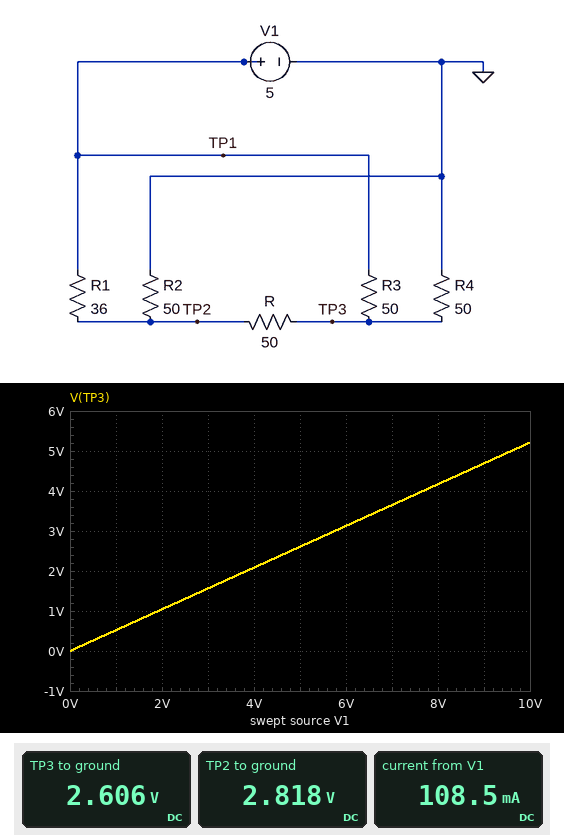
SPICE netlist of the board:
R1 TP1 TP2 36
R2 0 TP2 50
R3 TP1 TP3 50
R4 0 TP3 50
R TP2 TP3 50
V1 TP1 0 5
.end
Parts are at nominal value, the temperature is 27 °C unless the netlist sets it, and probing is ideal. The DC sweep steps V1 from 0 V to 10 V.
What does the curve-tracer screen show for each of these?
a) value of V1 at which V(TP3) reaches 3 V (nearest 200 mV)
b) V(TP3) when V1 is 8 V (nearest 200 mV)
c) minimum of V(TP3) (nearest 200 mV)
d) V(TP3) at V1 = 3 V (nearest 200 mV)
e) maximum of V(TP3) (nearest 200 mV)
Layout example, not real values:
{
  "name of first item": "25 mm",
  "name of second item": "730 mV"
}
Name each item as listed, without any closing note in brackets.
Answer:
{
  "value of V1 at which V(TP3) reaches 3 V": "5.8 V",
  "V(TP3) when V1 is 8 V": "4.2 V",
  "minimum of V(TP3)": "0 V",
  "V(TP3) at V1 = 3 V": "1.6 V",
  "maximum of V(TP3)": "5.2 V"
}
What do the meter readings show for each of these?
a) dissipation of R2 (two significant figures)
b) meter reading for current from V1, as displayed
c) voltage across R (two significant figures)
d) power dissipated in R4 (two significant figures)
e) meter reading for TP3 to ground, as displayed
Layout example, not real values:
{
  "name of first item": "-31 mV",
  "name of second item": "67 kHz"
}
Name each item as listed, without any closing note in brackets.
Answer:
{
  "dissipation of R2": "160 mW",
  "meter reading for current from V1, as displayed": "108.5 mA",
  "voltage across R": "210 mV",
  "power dissipated in R4": "140 mW",
  "meter reading for TP3 to ground, as displayed": "2.606 V"
}
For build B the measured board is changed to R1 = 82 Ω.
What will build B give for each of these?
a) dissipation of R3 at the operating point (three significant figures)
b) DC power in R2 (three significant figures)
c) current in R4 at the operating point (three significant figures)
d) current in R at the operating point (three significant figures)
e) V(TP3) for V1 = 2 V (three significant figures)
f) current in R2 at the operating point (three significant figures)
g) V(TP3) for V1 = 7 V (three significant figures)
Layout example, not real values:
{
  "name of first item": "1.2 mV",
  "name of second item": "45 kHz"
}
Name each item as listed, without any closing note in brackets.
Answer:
{
  "dissipation of R3 at the operating point": "140 mW",
  "DC power in R2": "85.8 mW",
  "current in R4 at the operating point": "47.1 mA",
  "current in R at the operating point": "5.71 mA",
  "V(TP3) for V1 = 2 V": "943 mV",
  "current in R2 at the operating point": "41.4 mA",
  "V(TP3) for V1 = 7 V": "3.30 V"
}
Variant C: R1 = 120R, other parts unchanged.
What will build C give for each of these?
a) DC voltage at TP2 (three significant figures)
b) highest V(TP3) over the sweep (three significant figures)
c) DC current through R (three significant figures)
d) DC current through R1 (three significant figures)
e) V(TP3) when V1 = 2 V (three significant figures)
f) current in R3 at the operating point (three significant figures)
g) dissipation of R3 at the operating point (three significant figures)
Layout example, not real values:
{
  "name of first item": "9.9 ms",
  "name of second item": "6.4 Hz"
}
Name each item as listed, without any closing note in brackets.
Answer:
{
  "DC voltage at TP2": "1.80 V",
  "highest V(TP3) over the sweep": "4.53 V",
  "DC current through R": "9.33 mA",
  "DC current through R1": "26.7 mA",
  "V(TP3) when V1 = 2 V": "907 mV",
  "current in R3 at the operating point": "54.7 mA",
  "dissipation of R3 at the operating point": "149 mW"
}
